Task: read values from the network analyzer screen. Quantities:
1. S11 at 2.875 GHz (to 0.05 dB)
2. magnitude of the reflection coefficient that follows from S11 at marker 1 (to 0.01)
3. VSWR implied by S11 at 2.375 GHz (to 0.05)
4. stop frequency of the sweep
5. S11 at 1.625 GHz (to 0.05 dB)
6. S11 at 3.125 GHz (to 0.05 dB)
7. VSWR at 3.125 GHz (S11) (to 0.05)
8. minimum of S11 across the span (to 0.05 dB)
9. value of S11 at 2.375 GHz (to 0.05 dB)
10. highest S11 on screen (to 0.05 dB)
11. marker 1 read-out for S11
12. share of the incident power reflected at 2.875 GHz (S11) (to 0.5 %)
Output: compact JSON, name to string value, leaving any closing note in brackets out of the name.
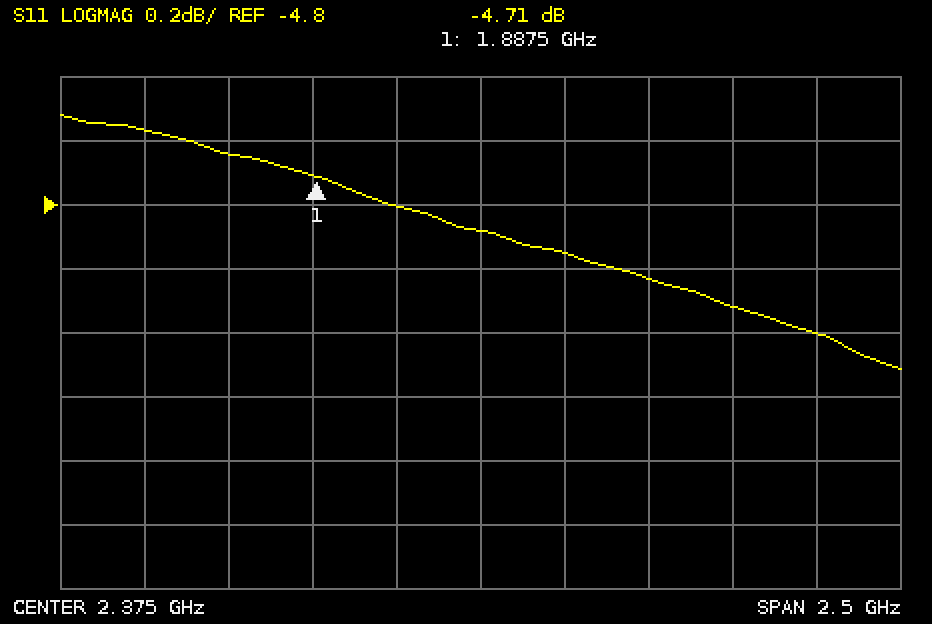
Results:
{"S11 at 2.875 GHz": "-5.05 dB", "magnitude of the reflection coefficient that follows from S11 at marker 1": "0.58", "VSWR implied by S11 at 2.375 GHz": "3.65", "stop frequency of the sweep": "3.625 GHz", "S11 at 1.625 GHz": "-4.65 dB", "S11 at 3.125 GHz": "-5.10 dB", "VSWR at 3.125 GHz (S11)": "3.50", "minimum of S11 across the span": "-5.30 dB", "value of S11 at 2.375 GHz": "-4.90 dB", "highest S11 on screen": "-4.50 dB", "marker 1 read-out for S11": "-4.71 dB", "share of the incident power reflected at 2.875 GHz (S11)": "31.5 %"}
